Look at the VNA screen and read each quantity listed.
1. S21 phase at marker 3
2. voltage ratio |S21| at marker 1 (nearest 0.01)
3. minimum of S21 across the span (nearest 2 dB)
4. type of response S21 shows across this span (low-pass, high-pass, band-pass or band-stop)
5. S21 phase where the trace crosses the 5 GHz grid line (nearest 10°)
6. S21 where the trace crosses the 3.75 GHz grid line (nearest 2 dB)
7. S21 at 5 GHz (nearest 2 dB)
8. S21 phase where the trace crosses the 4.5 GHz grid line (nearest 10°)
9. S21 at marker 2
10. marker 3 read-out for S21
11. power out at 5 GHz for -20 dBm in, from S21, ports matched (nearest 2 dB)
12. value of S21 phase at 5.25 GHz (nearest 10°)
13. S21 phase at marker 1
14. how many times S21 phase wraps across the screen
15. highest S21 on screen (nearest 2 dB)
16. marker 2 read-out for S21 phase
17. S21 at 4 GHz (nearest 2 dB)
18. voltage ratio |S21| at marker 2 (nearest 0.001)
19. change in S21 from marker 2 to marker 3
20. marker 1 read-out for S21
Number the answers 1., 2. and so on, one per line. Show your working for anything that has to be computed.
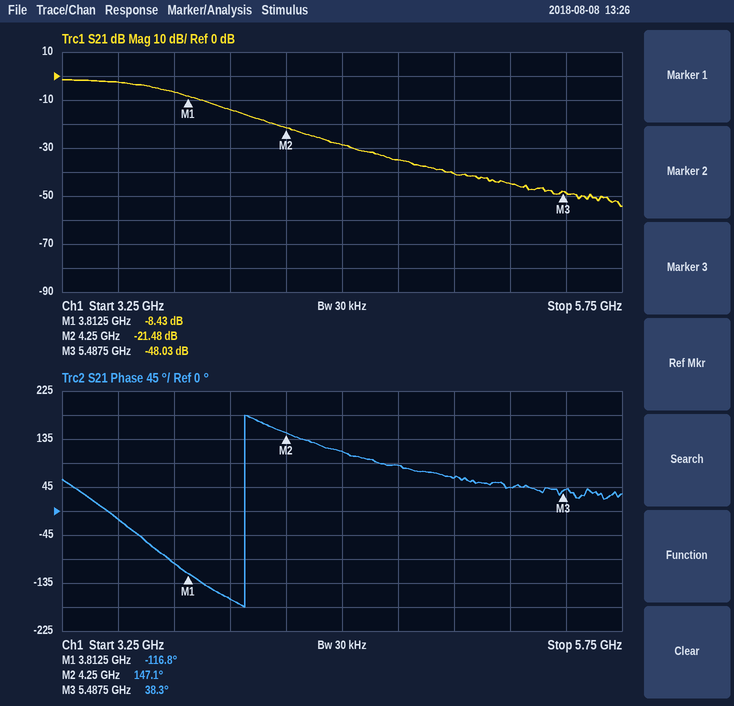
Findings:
1. 38.3°
2. 10^(-8.43/20) ≈ 0.38
3. -54 dB
4. low-pass
5. 60°
6. -6 dB
7. -40 dB
8. 110°
9. -21.48 dB
10. -48.03 dB
11. -20 dBm + (-40 dB) = -60 dBm
12. 40°
13. -116.8°
14. 1
15. -2 dB
16. 147.1°
17. -14 dB
18. 10^(-21.48/20) ≈ 0.084
19. -48.03 − (-21.48) = -26.55 dB
20. -8.43 dB
